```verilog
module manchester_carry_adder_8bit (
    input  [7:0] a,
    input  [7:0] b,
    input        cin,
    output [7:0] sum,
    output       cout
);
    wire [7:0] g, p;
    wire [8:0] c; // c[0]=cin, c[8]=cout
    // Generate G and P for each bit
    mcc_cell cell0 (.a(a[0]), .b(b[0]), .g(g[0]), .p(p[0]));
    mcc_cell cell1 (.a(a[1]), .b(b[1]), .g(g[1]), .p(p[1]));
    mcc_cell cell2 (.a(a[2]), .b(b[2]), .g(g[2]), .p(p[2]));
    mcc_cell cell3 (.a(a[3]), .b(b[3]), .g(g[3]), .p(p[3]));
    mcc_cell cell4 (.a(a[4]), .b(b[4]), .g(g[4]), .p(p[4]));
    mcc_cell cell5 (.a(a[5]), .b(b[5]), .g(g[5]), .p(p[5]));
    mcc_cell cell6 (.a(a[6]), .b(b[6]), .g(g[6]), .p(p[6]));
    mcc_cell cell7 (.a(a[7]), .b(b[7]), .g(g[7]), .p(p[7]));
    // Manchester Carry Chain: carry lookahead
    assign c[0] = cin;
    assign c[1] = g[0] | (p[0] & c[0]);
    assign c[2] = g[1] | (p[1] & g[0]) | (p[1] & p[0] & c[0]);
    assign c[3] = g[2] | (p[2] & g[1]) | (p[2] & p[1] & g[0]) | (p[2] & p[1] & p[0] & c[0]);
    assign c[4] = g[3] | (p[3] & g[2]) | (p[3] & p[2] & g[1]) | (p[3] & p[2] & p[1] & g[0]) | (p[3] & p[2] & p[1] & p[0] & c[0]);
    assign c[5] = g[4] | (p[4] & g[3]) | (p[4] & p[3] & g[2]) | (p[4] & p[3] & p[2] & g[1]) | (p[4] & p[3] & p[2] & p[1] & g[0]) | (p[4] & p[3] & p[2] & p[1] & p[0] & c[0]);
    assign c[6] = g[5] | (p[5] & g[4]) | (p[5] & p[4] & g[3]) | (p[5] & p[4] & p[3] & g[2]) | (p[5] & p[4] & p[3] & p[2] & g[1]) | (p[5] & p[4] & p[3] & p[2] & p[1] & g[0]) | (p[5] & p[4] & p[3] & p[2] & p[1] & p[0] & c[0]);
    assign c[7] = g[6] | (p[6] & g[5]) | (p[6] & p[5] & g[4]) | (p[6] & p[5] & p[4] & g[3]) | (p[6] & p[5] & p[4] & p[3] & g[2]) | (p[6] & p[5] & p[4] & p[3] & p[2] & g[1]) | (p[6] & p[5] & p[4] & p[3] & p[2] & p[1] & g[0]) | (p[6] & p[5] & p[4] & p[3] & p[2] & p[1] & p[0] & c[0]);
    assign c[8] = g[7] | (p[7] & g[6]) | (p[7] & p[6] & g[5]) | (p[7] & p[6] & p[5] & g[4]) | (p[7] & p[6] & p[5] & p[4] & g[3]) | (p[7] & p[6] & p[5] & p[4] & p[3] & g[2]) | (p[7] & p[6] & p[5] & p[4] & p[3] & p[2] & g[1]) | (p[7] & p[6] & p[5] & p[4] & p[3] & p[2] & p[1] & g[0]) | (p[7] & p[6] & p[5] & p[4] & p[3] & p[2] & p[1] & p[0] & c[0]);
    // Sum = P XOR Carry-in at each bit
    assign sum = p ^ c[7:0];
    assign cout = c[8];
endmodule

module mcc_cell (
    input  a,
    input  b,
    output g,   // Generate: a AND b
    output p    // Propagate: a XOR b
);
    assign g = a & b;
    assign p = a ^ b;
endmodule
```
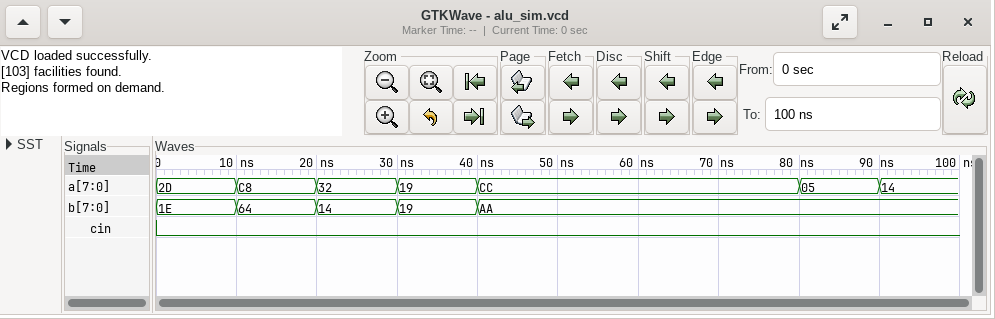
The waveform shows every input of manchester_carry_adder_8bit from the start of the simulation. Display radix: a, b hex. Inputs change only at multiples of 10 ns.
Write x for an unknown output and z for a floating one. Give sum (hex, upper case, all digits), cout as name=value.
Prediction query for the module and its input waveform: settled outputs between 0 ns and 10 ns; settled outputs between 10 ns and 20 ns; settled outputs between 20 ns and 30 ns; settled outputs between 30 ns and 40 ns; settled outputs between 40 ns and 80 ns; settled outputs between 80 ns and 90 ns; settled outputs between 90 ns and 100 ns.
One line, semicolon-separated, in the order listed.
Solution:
sum=4B, cout=0; sum=2C, cout=1; sum=46, cout=0; sum=32, cout=0; sum=76, cout=1; sum=AF, cout=0; sum=BE, cout=0
